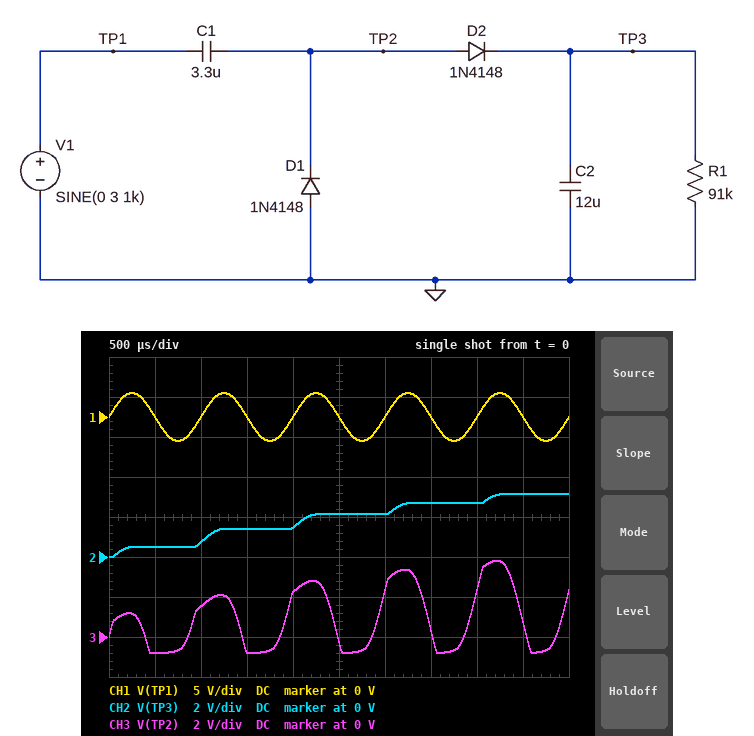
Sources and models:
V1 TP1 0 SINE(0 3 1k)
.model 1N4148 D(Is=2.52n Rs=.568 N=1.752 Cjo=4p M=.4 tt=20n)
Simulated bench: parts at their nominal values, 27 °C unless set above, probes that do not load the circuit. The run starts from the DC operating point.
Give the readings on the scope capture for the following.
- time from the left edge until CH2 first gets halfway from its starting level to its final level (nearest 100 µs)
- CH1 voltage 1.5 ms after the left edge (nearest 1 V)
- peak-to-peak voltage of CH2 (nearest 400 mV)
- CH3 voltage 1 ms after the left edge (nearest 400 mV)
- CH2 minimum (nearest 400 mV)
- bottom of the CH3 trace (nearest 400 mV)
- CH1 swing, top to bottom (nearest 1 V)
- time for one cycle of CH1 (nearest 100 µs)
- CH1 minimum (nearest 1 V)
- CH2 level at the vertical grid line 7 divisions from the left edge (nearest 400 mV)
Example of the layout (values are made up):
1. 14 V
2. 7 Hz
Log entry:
1. 2.0 ms
2. 0 V
3. 3.2 V
4. 1.6 V
5. 0 V
6. -800 mV
7. 6 V
8. 1.0 ms
9. -3 V
10. 2.8 V
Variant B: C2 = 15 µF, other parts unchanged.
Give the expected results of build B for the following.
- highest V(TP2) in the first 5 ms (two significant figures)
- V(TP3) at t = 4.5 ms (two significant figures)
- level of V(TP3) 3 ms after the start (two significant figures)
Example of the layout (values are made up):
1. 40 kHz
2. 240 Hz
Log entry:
1. 3.5 V
2. 2.8 V
3. 1.8 V
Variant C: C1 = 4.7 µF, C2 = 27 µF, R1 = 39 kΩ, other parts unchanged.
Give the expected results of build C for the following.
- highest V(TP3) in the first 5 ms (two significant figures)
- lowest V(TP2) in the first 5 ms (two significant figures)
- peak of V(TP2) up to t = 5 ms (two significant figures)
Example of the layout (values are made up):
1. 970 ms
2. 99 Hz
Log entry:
1. 2.4 V
2. -840 mV
3. 3.1 V
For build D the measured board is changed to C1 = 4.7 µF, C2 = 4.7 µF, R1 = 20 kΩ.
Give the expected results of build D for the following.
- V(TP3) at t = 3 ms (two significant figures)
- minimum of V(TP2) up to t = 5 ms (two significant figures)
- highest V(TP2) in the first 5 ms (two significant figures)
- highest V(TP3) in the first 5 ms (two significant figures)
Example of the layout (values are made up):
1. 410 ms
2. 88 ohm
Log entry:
1. 3.8 V
2. -840 mV
3. 5.1 V
4. 4.5 V
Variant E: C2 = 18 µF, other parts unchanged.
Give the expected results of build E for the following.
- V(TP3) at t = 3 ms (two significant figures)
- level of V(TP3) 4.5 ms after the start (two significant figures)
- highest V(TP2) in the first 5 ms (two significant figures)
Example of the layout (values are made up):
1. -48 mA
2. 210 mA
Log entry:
1. 1.6 V
2. 2.5 V
3. 3.2 V
